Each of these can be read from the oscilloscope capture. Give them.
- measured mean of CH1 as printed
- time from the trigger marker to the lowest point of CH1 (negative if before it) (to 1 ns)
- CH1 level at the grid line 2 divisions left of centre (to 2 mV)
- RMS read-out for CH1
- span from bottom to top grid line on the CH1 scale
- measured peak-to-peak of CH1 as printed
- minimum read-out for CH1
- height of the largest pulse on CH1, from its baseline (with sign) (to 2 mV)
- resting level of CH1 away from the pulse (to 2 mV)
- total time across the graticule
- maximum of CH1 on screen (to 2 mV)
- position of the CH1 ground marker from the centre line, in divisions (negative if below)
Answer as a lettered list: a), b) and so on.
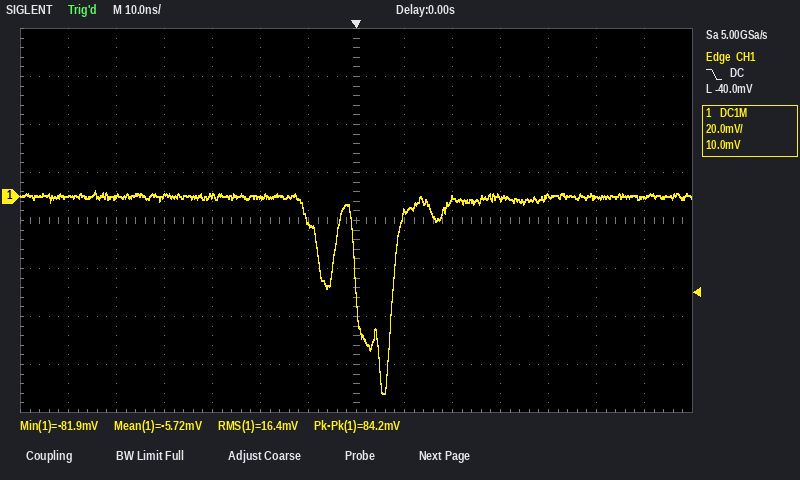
a) -5.72 mV
b) +6 ns
c) 0 mV
d) 16.4 mV
e) 160 mV
f) 84.2 mV
g) -81.9 mV
h) -82 mV
i) 0 mV
j) 140 ns
k) 2 mV
l) +0.5 div
